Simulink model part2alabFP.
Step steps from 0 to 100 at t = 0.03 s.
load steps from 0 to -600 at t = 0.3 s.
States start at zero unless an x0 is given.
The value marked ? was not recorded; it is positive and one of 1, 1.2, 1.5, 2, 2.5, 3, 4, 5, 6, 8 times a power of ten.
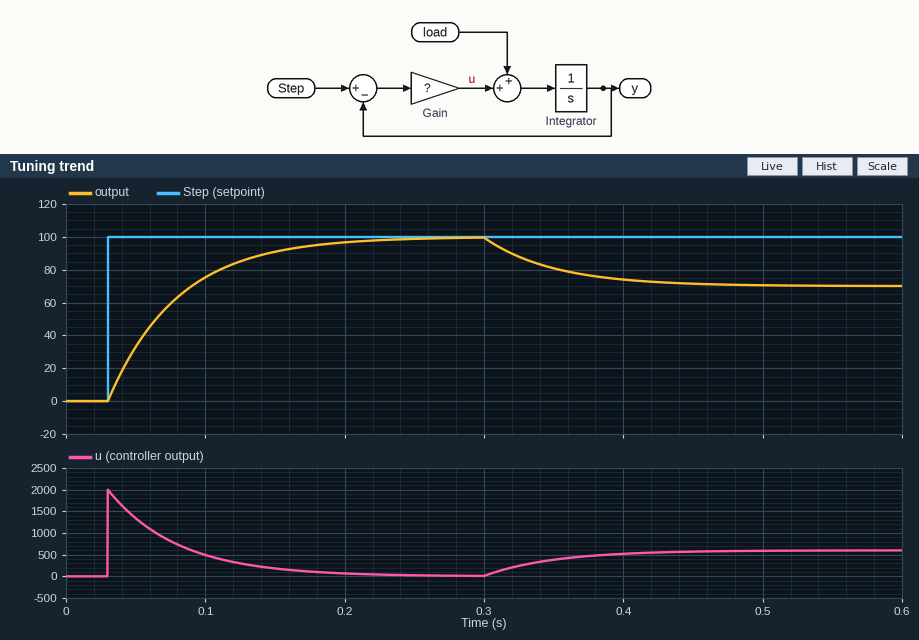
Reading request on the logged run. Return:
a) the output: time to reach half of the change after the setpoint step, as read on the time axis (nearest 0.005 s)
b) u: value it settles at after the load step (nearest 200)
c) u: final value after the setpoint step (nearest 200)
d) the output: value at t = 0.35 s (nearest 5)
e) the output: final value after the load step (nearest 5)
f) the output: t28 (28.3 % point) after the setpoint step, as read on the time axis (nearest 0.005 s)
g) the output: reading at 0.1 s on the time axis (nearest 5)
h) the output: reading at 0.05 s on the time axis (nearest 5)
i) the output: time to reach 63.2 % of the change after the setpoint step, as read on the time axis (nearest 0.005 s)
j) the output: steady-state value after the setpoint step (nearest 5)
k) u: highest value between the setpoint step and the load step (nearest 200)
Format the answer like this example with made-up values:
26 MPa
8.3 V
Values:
0.065 s
600
0
80
70
0.045 s
75
35
0.080 s
100
2000
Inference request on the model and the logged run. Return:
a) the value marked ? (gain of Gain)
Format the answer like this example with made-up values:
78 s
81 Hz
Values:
20
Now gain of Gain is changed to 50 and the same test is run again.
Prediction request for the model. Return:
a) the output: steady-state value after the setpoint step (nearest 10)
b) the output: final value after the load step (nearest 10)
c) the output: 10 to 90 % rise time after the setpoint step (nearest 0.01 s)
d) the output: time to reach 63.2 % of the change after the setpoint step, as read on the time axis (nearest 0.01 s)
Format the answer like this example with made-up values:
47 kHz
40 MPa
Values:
100
90
0.04 s
0.05 s
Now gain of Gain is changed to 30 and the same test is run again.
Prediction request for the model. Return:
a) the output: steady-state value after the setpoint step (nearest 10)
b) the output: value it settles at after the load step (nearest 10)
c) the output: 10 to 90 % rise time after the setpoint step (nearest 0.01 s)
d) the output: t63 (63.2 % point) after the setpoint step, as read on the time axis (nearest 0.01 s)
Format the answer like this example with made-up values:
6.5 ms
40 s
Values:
100
80
0.07 s
0.06 s
